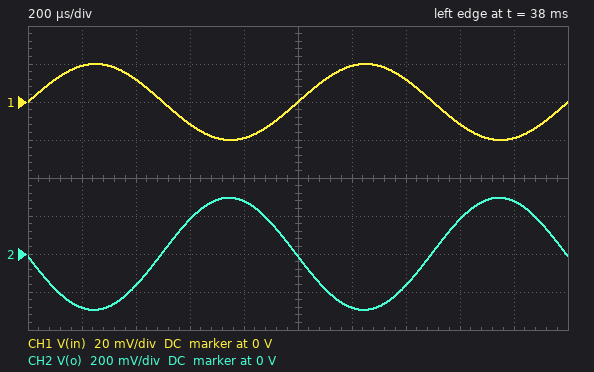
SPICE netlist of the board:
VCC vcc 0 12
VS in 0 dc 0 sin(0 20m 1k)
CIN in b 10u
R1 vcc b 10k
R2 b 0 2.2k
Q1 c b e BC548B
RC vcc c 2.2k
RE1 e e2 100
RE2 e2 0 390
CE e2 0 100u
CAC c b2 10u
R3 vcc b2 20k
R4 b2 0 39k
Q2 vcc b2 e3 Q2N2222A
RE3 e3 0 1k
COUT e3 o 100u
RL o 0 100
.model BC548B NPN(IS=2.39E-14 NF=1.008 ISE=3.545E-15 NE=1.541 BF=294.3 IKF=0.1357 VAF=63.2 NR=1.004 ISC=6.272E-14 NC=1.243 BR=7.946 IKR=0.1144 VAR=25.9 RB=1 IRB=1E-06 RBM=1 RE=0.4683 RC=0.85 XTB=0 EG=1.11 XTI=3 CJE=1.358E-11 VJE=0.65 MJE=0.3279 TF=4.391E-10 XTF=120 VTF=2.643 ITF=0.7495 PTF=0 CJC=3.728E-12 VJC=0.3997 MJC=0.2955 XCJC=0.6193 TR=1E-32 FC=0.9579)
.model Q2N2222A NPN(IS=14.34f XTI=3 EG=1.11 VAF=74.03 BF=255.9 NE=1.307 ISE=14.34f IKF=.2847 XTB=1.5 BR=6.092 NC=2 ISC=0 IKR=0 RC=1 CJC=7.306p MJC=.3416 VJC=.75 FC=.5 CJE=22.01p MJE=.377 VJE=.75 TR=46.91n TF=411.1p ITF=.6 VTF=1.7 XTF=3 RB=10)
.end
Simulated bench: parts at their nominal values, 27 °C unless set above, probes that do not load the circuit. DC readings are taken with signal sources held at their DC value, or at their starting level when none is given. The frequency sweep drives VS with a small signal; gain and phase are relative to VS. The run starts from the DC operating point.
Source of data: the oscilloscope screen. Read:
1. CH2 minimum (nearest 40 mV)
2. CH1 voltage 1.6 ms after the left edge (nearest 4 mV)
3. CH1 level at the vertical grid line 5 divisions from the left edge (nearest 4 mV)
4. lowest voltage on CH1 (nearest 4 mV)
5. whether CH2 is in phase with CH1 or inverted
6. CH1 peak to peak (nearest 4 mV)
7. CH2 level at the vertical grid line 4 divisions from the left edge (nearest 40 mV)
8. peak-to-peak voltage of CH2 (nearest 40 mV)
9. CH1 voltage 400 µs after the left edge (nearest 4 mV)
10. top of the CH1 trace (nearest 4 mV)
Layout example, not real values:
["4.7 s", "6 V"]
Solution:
["-280 mV", "-12 mV", "0 V", "-20 mV", "inverted", "40 mV", "280 mV", "600 mV", "12 mV", "20 mV"]
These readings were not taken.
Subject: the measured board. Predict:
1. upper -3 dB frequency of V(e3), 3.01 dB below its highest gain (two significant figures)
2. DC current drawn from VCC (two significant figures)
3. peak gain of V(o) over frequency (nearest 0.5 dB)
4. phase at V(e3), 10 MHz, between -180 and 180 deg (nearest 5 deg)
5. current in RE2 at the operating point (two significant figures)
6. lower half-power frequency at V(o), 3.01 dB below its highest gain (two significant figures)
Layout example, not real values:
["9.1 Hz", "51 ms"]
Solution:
["7.9 MHz", "11 mA", "23.5 dB", "125 deg", "3.0 mA", "28 Hz"]
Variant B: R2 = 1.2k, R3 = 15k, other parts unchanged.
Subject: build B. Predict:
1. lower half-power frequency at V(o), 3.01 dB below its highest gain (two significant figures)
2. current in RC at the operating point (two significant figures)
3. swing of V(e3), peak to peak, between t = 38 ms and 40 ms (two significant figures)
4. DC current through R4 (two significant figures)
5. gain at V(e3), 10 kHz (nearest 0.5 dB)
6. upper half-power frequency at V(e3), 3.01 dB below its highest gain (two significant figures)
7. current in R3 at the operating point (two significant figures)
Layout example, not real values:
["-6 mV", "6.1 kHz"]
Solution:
["31 Hz", "1.3 mA", "520 mV", "210 µA", "22.5 dB", "8.4 MHz", "250 µA"]
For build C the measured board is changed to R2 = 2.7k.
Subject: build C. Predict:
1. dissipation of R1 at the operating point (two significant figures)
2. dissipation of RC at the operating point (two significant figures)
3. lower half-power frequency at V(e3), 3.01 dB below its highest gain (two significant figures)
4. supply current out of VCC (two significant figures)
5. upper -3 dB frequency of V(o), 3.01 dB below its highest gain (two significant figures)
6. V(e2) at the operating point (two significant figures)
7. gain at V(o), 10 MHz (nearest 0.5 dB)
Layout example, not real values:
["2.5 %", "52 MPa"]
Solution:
["9.0 mW", "31 mW", "20 Hz", "12 mA", "7.6 MHz", "1.5 V", "19.0 dB"]
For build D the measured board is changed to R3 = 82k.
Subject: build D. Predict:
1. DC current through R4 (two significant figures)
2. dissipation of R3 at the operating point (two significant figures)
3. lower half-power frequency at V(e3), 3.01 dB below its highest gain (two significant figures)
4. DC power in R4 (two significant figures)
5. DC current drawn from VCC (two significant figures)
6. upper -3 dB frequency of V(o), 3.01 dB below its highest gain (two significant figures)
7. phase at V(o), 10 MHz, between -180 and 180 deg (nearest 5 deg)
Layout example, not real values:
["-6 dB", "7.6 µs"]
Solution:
["89 µA", "890 µW", "20 Hz", "310 µW", "6.9 mA", "6.8 MHz", "120 deg"]
